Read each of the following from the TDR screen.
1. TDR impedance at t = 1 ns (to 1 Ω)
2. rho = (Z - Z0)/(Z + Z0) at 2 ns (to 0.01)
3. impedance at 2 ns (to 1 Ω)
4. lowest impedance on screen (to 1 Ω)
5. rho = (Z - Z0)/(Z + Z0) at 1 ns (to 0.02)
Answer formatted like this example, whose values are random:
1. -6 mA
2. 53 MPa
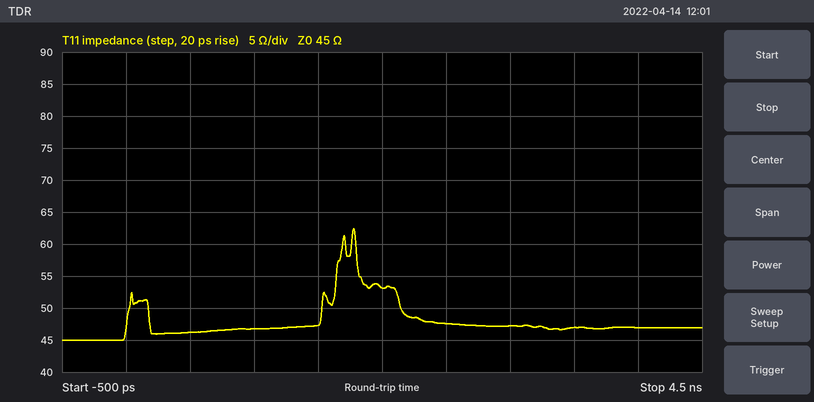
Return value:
1. 47 Ω
2. +0.08
3. 53 Ω
4. 45 Ω
5. +0.02
